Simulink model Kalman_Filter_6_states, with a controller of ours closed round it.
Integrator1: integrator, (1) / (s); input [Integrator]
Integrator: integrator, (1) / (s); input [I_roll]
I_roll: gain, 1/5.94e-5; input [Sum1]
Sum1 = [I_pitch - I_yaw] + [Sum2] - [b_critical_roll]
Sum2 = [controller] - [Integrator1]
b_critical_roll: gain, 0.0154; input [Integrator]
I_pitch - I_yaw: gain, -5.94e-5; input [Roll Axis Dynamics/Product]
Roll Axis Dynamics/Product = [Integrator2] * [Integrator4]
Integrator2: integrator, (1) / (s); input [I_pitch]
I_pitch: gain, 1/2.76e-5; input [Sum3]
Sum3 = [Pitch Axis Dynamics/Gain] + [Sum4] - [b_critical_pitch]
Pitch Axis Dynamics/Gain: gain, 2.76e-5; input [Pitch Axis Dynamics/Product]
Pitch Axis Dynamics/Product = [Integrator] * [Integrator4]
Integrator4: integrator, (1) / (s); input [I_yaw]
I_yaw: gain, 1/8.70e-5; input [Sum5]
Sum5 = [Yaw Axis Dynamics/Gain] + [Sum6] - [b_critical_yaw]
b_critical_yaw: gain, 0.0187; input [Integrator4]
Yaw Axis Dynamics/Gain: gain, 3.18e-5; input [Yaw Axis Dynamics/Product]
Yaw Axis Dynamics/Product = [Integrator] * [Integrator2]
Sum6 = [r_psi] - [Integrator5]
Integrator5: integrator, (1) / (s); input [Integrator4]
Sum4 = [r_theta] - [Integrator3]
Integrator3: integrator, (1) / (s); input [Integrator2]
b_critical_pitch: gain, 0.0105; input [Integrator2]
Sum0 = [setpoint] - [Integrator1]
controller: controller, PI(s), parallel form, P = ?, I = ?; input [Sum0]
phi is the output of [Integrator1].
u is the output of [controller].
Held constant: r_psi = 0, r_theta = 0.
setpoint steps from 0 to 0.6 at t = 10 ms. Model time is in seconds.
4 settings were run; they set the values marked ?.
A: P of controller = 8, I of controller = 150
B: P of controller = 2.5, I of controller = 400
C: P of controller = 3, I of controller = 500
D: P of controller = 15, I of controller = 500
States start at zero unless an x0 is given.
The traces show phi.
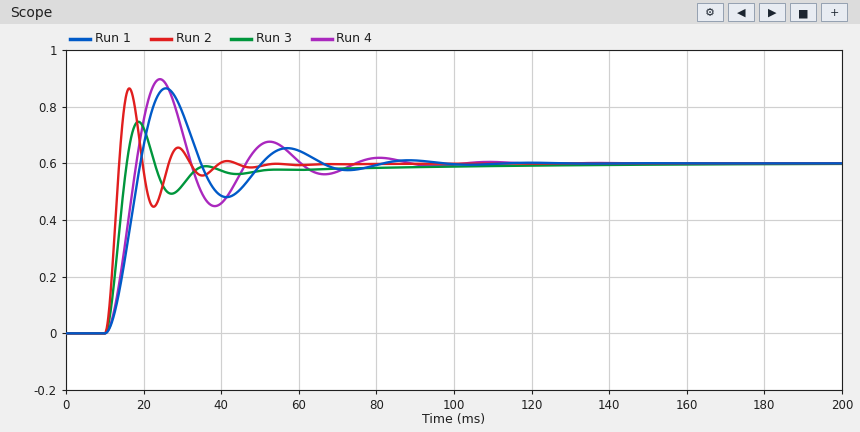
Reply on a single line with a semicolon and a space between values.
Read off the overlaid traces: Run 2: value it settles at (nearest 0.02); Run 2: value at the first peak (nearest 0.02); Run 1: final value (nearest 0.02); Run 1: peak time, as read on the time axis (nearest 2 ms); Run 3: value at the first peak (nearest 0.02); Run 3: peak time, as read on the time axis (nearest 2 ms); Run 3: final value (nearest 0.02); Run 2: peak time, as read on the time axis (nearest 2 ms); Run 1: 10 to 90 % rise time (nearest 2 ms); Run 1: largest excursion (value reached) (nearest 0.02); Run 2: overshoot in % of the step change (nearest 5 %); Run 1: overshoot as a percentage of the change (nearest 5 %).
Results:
0.60; 0.86; 0.60; 26 ms; 0.74; 18 ms; 0.60; 16 ms; 6 ms; 0.86; 45 %; 45 %
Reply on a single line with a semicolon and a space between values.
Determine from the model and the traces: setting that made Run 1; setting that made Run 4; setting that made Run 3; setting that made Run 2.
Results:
B; C; A; D
